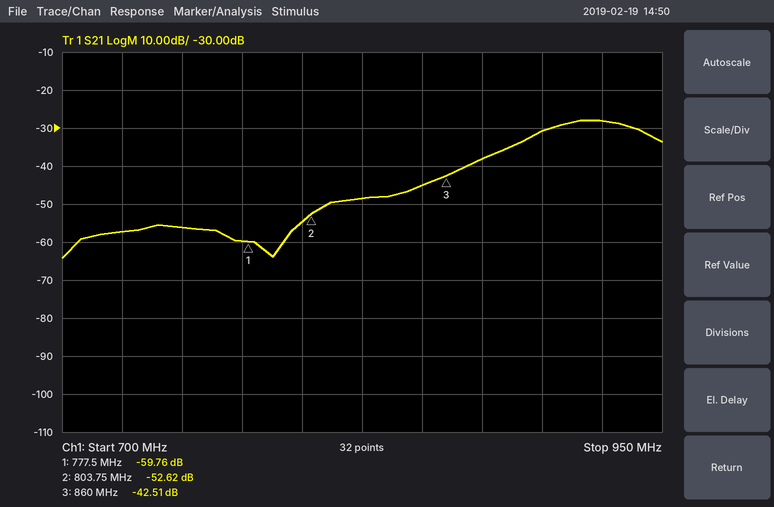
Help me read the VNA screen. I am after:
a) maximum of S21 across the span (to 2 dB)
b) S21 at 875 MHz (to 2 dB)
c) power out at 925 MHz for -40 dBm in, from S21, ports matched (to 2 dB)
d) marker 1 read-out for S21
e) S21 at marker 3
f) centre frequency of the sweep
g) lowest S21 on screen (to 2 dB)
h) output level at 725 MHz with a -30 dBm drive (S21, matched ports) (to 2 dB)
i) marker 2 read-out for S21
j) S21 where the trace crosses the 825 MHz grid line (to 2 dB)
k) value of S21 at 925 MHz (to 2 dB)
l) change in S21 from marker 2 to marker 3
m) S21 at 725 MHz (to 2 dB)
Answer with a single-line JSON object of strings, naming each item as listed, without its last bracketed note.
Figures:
{"maximum of S21 across the span": "-28 dB", "S21 at 875 MHz": "-38 dB", "power out at 925 MHz for -40 dBm in, from S21, ports matched": "-68 dBm", "marker 1 read-out for S21": "-59.76 dB", "S21 at marker 3": "-42.51 dB", "centre frequency of the sweep": "825 MHz", "lowest S21 on screen": "-64 dB", "output level at 725 MHz with a -30 dBm drive (S21, matched ports)": "-88 dBm", "marker 2 read-out for S21": "-52.62 dB", "S21 where the trace crosses the 825 MHz grid line": "-48 dB", "value of S21 at 925 MHz": "-28 dB", "change in S21 from marker 2 to marker 3": "10.11 dB", "S21 at 725 MHz": "-58 dB"}
